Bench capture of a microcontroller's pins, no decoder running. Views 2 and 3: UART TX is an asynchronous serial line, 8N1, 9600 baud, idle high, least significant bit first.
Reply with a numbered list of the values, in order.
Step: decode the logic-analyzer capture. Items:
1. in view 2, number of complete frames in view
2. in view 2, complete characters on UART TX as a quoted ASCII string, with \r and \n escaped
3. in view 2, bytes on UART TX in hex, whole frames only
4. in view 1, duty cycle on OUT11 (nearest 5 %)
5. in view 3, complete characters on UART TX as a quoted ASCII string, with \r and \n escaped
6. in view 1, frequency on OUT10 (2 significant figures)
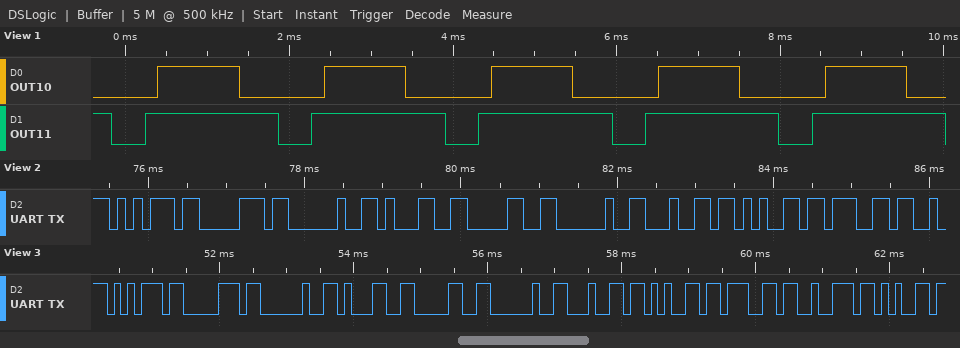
1. 9
2. "up 10 deg"
3. 75 70 20 31 30 20 64 65 67
4. 80 %
5. "up 10 degre"
6. 490 Hz
